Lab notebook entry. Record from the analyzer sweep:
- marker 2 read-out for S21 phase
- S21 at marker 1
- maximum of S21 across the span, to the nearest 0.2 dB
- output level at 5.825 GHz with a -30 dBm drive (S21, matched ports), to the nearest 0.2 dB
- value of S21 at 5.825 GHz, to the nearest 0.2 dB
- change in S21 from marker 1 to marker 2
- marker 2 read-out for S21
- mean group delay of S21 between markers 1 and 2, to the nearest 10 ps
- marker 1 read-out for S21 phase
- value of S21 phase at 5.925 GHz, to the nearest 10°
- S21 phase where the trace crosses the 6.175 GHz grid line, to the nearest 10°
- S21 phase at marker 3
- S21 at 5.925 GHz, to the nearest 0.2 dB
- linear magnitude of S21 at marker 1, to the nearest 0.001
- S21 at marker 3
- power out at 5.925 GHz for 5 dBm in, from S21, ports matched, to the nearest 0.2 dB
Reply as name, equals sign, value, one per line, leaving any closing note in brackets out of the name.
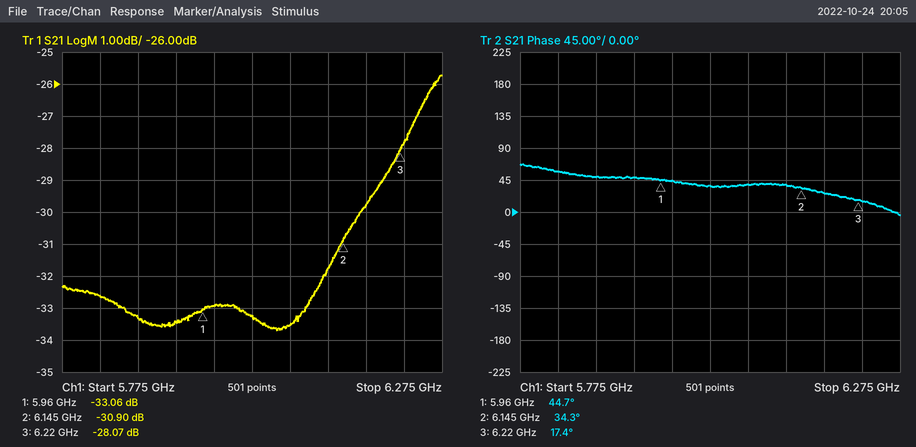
marker 2 read-out for S21 phase = 34.3°
S21 at marker 1 = -33.06 dB
maximum of S21 across the span, to the nearest 0.2 dB = -25.8 dB
output level at 5.825 GHz with a -30 dBm drive (S21, matched ports), to the nearest 0.2 dB = -62.6 dBm
value of S21 at 5.825 GHz, to the nearest 0.2 dB = -32.6 dB
change in S21 from marker 1 to marker 2 = 2.16 dB
marker 2 read-out for S21 = -30.90 dB
mean group delay of S21 between markers 1 and 2, to the nearest 10 ps = 160 ps
marker 1 read-out for S21 phase = 44.7°
value of S21 phase at 5.925 GHz, to the nearest 10° = 50°
S21 phase where the trace crosses the 6.175 GHz grid line, to the nearest 10° = 30°
S21 phase at marker 3 = 17.4°
S21 at 5.925 GHz, to the nearest 0.2 dB = -33.4 dB
linear magnitude of S21 at marker 1, to the nearest 0.001 = 0.022
S21 at marker 3 = -28.07 dB
power out at 5.925 GHz for 5 dBm in, from S21, ports matched, to the nearest 0.2 dB = -28.4 dBm
